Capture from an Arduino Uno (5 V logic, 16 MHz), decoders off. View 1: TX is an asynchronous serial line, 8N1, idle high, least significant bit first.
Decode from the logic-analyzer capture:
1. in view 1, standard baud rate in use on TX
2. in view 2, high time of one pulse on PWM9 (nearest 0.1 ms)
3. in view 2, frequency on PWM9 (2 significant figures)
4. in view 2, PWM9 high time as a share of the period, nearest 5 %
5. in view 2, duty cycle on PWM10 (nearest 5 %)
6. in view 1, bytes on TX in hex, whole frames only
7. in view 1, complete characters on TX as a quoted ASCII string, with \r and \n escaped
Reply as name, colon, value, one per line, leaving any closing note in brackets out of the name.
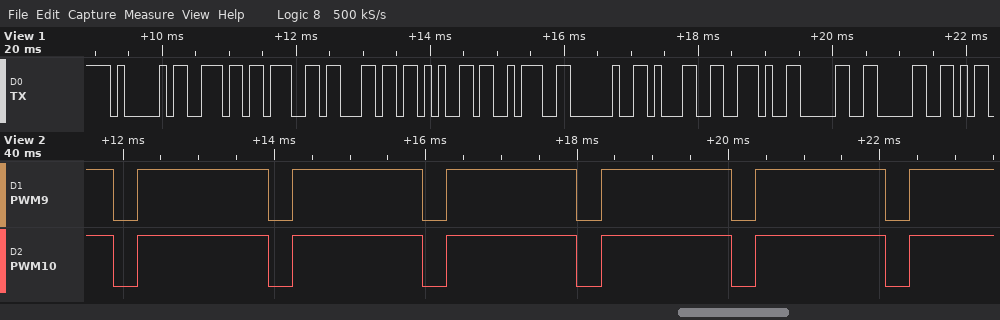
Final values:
in view 1, standard baud rate in use on TX: 9600 baud
in view 2, high time of one pulse on PWM9: 1.7 ms
in view 2, frequency on PWM9: 490 Hz
in view 2, PWM9 high time as a share of the period, nearest 5 %: 85 %
in view 2, duty cycle on PWM10: 85 %
in view 1, bytes on TX in hex, whole frames only: 41 6E 67 6C 65 3A 20 31 2E 30 30
in view 1, complete characters on TX as a quoted ASCII string, with \r and \n escaped: "Angle: 1.00"
